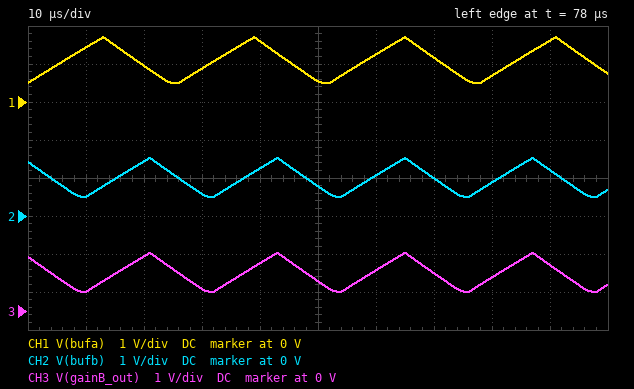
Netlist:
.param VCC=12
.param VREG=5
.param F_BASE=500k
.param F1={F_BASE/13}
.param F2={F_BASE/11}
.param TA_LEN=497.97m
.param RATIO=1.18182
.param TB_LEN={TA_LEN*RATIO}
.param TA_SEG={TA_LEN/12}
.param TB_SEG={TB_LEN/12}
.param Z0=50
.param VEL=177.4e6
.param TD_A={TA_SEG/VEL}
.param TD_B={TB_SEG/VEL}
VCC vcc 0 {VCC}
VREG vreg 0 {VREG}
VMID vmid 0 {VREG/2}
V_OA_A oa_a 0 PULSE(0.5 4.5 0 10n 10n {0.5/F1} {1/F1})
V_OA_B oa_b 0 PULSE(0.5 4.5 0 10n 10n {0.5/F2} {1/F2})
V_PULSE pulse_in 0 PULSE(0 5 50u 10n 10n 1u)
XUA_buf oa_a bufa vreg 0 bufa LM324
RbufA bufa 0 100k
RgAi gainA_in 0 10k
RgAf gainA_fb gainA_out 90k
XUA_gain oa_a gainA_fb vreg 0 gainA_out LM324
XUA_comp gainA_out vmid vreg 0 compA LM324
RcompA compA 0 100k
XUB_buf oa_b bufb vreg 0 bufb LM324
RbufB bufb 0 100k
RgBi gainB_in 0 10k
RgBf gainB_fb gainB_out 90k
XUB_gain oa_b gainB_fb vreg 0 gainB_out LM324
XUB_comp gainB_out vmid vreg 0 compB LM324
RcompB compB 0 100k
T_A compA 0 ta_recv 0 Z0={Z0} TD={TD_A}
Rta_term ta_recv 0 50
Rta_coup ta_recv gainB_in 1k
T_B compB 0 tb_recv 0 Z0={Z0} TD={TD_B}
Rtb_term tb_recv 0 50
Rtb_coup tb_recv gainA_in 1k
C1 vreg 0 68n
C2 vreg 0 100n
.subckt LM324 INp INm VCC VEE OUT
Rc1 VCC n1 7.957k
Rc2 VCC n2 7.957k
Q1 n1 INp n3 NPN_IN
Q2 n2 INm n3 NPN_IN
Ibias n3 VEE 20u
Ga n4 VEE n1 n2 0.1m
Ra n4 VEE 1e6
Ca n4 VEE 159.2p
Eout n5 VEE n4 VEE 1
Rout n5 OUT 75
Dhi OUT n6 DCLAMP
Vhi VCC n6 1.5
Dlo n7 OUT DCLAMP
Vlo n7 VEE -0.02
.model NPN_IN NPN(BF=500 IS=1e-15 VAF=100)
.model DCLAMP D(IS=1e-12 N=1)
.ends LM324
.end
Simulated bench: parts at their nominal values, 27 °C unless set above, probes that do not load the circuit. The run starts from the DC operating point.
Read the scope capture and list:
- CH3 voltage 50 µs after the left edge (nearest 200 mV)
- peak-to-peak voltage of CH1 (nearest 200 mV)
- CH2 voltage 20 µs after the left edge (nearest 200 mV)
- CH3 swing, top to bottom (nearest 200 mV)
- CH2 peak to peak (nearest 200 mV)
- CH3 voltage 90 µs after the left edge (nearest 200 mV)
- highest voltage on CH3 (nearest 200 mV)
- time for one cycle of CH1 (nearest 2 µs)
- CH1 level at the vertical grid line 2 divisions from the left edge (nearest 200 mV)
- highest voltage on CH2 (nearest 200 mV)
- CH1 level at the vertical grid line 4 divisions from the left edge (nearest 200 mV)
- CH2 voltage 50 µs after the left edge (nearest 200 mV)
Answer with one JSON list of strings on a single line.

["800 mV", "1.2 V", "1.4 V", "1.0 V", "1.0 V", "1.2 V", "1.6 V", "26 µs", "1.0 V", "1.6 V", "1.6 V", "800 mV"]
